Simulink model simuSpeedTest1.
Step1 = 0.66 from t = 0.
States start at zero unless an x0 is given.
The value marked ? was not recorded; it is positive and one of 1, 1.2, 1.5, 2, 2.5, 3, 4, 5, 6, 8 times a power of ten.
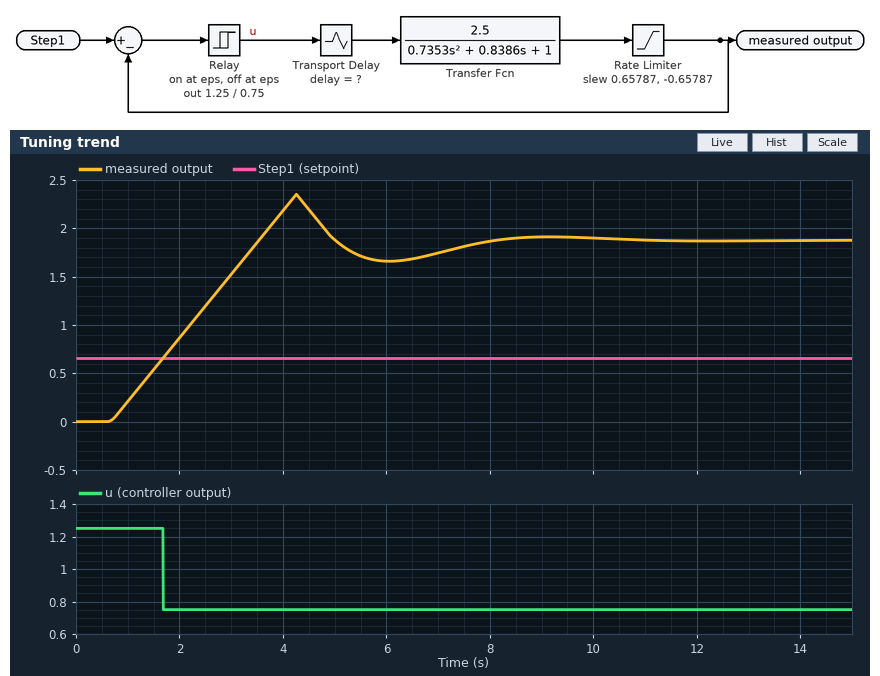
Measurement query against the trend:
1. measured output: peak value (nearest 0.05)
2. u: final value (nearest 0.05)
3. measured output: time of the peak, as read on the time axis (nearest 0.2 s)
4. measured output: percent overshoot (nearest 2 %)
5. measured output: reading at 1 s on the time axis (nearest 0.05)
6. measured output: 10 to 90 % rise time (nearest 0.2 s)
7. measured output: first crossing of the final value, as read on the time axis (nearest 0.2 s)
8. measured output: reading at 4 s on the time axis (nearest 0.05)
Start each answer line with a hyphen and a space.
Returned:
- 2.35
- 0.75
- 4.2 s
- 26 %
- 0.20
- 2.2 s
- 3.6 s
- 2.20
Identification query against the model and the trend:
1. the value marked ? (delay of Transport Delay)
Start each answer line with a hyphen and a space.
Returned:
- 0.6
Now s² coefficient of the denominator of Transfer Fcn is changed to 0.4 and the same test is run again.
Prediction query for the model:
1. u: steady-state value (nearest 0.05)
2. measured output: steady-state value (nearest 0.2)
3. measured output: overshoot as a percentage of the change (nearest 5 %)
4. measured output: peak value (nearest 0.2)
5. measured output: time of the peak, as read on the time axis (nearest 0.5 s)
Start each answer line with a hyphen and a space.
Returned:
- 0.75
- 1.8
- 15 %
- 2.2
- 4.0 s
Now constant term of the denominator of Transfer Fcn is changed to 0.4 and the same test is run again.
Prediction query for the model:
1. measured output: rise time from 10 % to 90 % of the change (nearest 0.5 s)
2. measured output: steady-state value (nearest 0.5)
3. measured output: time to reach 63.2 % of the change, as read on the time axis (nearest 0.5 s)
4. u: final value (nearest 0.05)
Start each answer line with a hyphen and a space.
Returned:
- 5.5 s
- 4.5
- 5.0 s
- 0.75
